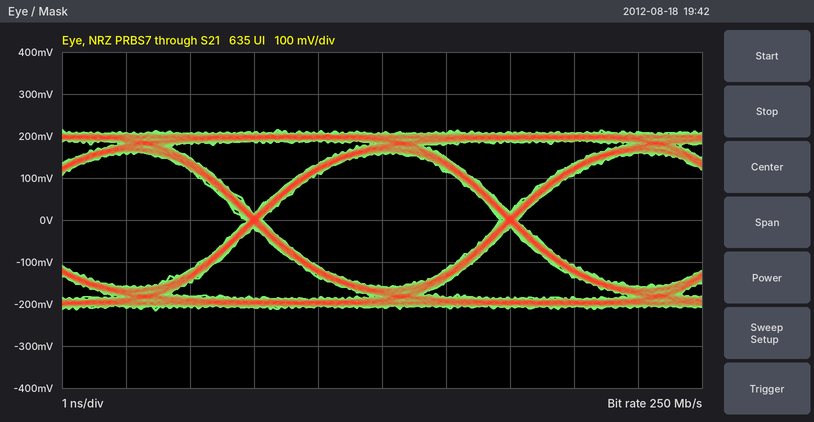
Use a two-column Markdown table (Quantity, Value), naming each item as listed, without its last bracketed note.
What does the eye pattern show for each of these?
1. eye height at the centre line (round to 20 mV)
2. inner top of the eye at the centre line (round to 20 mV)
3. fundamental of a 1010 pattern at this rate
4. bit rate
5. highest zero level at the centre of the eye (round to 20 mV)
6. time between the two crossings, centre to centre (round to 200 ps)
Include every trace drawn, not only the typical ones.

| Quantity | Value |
|---|---|
| eye height at the centre line | 320 mV |
| inner top of the eye at the centre line | 160 mV |
| fundamental of a 1010 pattern at this rate | 125 MHz |
| bit rate | 250 Mb/s |
| highest zero level at the centre of the eye | -160 mV |
| time between the two crossings, centre to centre | 4.0 ns |
